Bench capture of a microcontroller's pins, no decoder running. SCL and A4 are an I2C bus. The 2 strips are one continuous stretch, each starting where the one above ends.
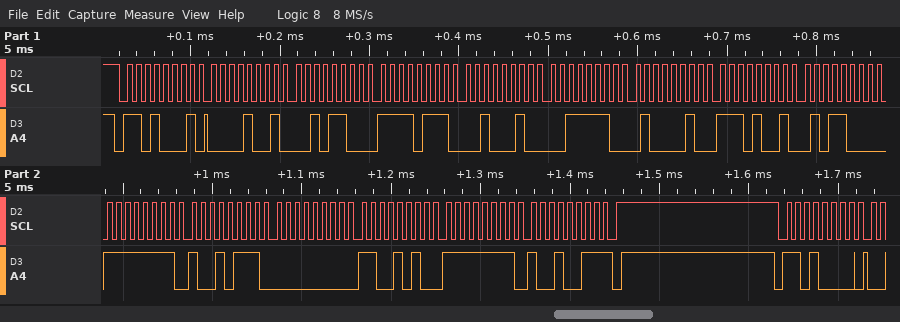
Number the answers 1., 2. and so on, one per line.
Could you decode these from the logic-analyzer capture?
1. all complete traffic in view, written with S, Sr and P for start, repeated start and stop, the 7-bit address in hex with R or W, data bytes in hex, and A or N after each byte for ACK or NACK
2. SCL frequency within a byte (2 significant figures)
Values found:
1. S 68R A 09 A 2C A F7 A 22 A 3E A 42 A E9 A 58 A FF A 97 A 00 A CA A FF A 93 N P S 68W A
2. 100 kHz
